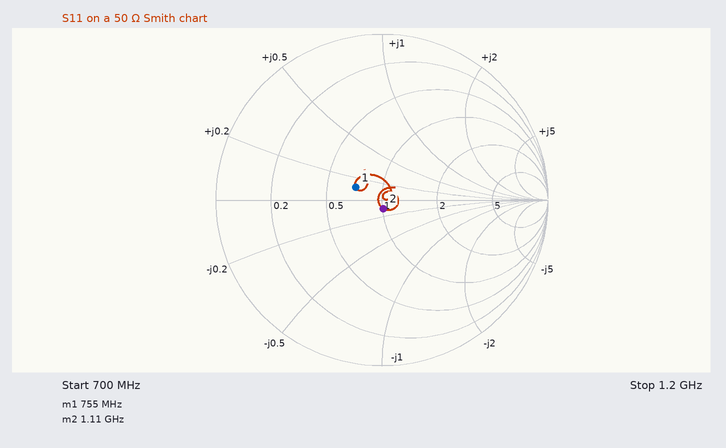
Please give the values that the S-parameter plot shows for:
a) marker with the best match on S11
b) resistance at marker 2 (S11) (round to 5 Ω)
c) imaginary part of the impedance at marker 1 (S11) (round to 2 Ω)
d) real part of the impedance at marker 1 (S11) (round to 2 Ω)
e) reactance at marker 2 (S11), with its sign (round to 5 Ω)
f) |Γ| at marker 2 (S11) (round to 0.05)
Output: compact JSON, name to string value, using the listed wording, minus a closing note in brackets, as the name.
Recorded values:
{"marker with the best match on S11": "marker 2", "resistance at marker 2 (S11)": "50 Ω", "imaginary part of the impedance at marker 1 (S11)": "+6 Ω", "real part of the impedance at marker 1 (S11)": "36 Ω", "reactance at marker 2 (S11), with its sign": "-5 Ω", "|Γ| at marker 2 (S11)": "0.05"}
